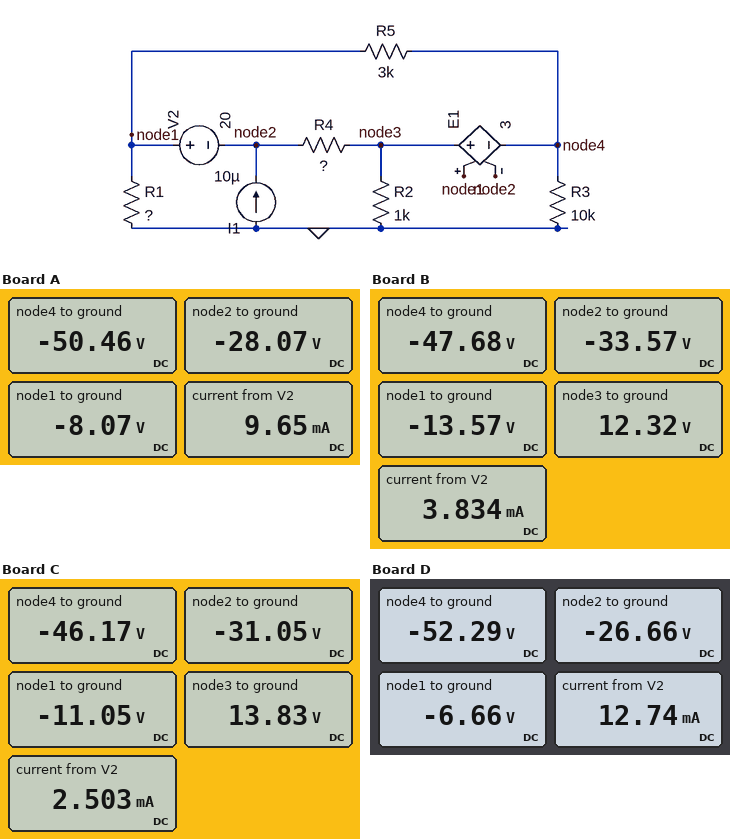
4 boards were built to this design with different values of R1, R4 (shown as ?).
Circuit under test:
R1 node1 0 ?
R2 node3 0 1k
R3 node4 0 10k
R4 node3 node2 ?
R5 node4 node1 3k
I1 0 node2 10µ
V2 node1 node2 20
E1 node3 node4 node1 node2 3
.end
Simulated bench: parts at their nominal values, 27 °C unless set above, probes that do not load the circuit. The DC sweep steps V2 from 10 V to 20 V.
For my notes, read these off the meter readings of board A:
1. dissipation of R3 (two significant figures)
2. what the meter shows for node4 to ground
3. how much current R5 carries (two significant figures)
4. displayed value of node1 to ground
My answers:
250 mW
-50.46 V
14 mA
-8.07 V
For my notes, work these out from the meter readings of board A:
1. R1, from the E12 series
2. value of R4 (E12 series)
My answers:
1.8 kΩ
3.9 kΩ
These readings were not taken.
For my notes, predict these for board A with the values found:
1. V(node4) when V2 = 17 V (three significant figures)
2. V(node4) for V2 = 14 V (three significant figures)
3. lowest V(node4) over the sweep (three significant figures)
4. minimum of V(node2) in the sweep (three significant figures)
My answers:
-42.9 V
-35.3 V
-50.5 V
-28.1 V
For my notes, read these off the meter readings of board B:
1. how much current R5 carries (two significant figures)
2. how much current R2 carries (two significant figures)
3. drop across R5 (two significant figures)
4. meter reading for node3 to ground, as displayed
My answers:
11 mA
12 mA
34 V
12.32 V
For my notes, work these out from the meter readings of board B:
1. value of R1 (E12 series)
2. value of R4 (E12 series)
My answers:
1.8 kΩ
12 kΩ
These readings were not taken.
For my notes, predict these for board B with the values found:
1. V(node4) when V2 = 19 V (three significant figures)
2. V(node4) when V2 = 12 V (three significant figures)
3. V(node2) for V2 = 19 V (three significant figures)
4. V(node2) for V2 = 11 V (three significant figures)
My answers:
-45.3 V
-28.6 V
-31.9 V
-18.5 V
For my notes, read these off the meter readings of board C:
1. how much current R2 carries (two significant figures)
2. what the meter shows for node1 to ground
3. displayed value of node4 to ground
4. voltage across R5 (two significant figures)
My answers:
14 mA
-11.05 V
-46.17 V
35 V
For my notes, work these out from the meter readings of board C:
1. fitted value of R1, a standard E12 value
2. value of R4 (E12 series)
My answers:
1.2 kΩ
18 kΩ
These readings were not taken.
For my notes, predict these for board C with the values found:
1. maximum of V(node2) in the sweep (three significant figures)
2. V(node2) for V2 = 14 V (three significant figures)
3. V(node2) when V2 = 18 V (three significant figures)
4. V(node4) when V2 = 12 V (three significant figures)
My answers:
-15.5 V
-21.7 V
-27.9 V
-27.7 V
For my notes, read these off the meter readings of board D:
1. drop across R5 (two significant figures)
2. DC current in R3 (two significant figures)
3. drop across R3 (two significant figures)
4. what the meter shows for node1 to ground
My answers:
46 V
5.2 mA
52 V
-6.66 V
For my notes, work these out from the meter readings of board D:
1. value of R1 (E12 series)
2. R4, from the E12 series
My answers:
2.7 kΩ
2.7 kΩ
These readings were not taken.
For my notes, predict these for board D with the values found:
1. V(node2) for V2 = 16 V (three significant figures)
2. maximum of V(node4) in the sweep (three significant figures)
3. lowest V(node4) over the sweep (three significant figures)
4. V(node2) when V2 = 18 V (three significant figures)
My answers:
-21.3 V
-26.1 V
-52.3 V
-24.0 V
